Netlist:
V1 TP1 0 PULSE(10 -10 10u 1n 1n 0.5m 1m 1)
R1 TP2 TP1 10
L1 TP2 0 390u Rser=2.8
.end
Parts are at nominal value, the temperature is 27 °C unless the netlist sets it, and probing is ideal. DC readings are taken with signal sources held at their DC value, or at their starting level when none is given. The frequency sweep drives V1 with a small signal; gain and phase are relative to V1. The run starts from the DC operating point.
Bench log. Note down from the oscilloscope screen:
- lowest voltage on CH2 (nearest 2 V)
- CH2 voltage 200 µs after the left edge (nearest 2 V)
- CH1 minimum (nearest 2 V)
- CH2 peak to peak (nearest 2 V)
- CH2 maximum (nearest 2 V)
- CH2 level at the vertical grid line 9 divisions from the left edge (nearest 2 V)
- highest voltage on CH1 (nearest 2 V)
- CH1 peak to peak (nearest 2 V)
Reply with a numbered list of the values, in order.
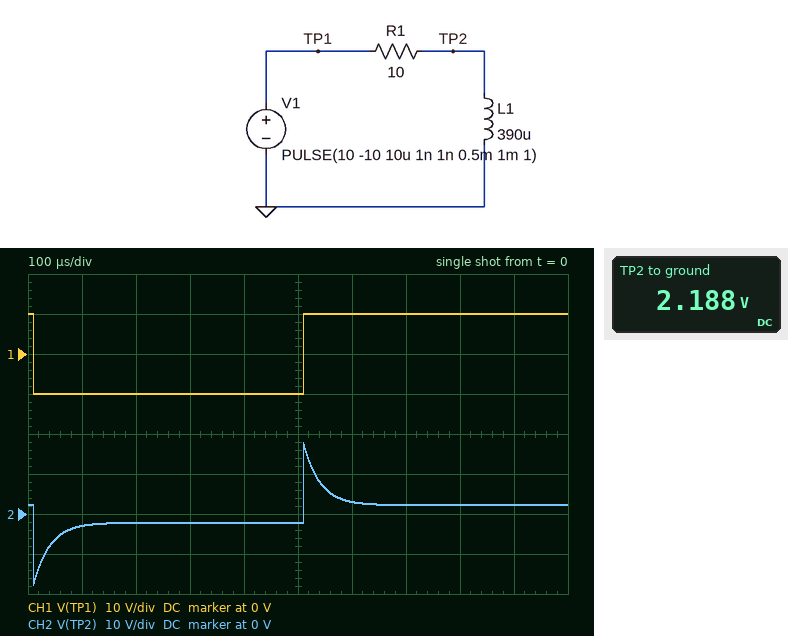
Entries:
1. -18 V
2. -2 V
3. -10 V
4. 36 V
5. 18 V
6. 2 V
7. 10 V
8. 20 V
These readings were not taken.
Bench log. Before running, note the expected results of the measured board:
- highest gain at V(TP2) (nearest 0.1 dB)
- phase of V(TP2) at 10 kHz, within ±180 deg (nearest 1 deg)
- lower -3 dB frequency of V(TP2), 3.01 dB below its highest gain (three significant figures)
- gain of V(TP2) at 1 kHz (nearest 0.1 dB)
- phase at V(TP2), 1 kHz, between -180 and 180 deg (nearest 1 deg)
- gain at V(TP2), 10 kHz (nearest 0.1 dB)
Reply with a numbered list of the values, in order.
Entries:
1. 0 dB
2. 21 deg
3. 4.97 kHz
4. -10.9 dB
5. 30 deg
6. -1.0 dB
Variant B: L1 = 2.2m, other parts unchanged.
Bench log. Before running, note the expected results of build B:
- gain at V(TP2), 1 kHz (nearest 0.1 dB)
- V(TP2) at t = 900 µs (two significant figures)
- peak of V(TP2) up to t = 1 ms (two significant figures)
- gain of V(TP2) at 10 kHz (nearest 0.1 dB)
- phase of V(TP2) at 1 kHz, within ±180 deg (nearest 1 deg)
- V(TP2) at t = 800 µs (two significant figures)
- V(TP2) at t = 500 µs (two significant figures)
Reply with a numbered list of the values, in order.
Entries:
1. -2.5 dB
2. 3.7 V
3. 17 V
4. 0 dB
5. 31 deg
6. 4.9 V
7. -3.1 V
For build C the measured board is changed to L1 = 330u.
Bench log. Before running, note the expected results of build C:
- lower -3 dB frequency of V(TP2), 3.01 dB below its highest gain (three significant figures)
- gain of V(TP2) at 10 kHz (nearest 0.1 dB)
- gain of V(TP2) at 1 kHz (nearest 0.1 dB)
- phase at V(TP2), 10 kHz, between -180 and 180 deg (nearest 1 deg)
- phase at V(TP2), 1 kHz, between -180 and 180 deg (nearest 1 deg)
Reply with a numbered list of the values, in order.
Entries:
1. 5.87 kHz
2. -1.3 dB
3. -11.4 dB
4. 24 deg
5. 27 deg
